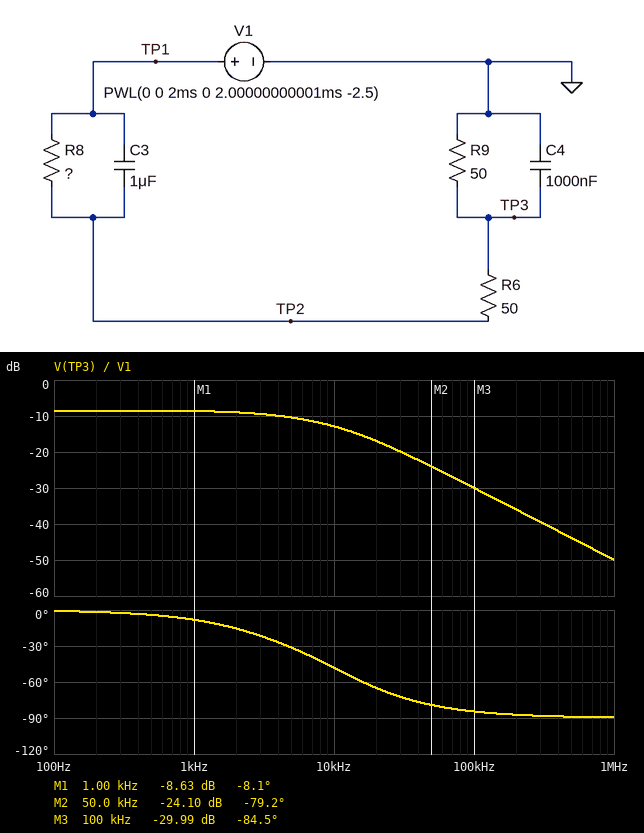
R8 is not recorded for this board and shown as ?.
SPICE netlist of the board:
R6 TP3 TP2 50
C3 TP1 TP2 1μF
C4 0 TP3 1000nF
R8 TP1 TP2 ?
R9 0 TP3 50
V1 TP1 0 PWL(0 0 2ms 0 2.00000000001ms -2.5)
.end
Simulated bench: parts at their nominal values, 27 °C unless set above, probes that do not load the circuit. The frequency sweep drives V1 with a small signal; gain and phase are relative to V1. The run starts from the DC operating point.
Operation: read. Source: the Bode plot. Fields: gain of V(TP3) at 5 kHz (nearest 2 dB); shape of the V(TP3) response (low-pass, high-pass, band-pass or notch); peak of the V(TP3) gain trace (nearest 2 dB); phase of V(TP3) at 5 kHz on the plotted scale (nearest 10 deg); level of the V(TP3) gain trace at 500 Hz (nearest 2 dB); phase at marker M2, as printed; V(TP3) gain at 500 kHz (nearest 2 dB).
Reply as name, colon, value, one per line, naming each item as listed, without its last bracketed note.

gain of V(TP3) at 5 kHz: -10 dB
shape of the V(TP3) response: low-pass
peak of the V(TP3) gain trace: -8 dB
phase of V(TP3) at 5 kHz on the plotted scale: -30 deg
level of the V(TP3) gain trace at 500 Hz: -8 dB
phase at marker M2, as printed: -79.2 deg
V(TP3) gain at 500 kHz: -44 dB
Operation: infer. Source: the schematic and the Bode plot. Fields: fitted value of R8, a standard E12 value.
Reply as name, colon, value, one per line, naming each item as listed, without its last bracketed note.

fitted value of R8, a standard E12 value: 33 Ω
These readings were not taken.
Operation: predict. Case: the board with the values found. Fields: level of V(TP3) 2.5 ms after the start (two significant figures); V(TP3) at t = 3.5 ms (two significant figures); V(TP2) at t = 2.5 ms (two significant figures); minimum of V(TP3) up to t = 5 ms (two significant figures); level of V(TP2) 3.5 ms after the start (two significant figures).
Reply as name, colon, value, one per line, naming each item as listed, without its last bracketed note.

level of V(TP3) 2.5 ms after the start: -940 mV
V(TP3) at t = 3.5 ms: -940 mV
V(TP2) at t = 2.5 ms: -1.9 V
minimum of V(TP3) up to t = 5 ms: -940 mV
level of V(TP2) 3.5 ms after the start: -1.9 V
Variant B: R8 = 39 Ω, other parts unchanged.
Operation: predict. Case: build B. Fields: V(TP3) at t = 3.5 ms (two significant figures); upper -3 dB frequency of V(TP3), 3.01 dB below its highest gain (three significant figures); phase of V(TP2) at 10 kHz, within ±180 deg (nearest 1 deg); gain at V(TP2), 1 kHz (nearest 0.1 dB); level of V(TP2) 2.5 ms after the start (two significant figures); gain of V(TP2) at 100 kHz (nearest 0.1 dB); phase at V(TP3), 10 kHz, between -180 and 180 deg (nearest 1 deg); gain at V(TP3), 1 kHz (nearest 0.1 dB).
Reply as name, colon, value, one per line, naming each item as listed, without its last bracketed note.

V(TP3) at t = 3.5 ms: -900 mV
upper -3 dB frequency of V(TP3), 3.01 dB below its highest gain: 7.97 kHz
phase of V(TP2) at 10 kHz, within ±180 deg: 10 deg
gain at V(TP2), 1 kHz: -2.9 dB
level of V(TP2) 2.5 ms after the start: -1.8 V
gain of V(TP2) at 100 kHz: 0 dB
phase at V(TP3), 10 kHz, between -180 and 180 deg: -47 deg
gain at V(TP3), 1 kHz: -9.0 dB
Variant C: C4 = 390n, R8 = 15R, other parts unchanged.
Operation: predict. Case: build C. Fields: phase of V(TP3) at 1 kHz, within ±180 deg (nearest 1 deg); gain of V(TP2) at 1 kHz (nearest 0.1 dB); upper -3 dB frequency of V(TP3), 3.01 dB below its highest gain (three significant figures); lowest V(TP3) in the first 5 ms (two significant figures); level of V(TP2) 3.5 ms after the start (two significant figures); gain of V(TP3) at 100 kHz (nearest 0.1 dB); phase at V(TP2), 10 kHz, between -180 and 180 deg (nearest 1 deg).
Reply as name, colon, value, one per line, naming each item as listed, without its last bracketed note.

phase of V(TP3) at 1 kHz, within ±180 deg: -3 deg
gain of V(TP2) at 1 kHz: -1.2 dB
upper -3 dB frequency of V(TP3), 3.01 dB below its highest gain: 17.9 kHz
lowest V(TP3) in the first 5 ms: -1.1 V
level of V(TP2) 3.5 ms after the start: -2.2 V
gain of V(TP3) at 100 kHz: -21.9 dB
phase at V(TP2), 10 kHz, between -180 and 180 deg: 3 deg
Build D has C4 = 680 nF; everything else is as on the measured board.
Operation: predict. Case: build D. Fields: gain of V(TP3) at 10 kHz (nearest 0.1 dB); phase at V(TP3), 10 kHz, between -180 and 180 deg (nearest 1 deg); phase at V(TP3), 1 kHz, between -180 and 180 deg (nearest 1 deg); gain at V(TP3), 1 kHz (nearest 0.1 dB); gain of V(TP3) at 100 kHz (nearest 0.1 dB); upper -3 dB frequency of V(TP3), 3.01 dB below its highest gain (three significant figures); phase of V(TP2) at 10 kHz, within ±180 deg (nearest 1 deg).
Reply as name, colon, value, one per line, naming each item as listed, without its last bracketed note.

gain of V(TP3) at 10 kHz: -10.7 dB
phase at V(TP3), 10 kHz, between -180 and 180 deg: -39 deg
phase at V(TP3), 1 kHz, between -180 and 180 deg: -5 deg
gain at V(TP3), 1 kHz: -8.5 dB
gain of V(TP3) at 100 kHz: -26.7 dB
upper -3 dB frequency of V(TP3), 3.01 dB below its highest gain: 12.3 kHz
phase of V(TP2) at 10 kHz, within ±180 deg: 8 deg
